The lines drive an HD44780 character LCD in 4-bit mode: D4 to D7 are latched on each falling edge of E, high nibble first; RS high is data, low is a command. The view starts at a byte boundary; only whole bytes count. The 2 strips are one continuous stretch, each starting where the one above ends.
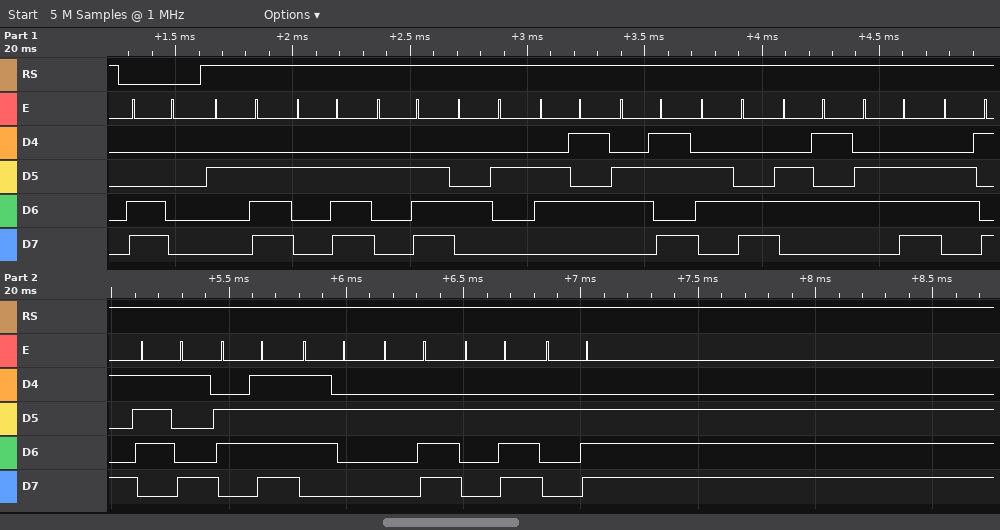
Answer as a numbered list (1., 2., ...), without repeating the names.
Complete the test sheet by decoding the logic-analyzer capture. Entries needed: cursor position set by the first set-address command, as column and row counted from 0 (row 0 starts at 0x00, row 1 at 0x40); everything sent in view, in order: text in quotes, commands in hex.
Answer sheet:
1. column 0, row 1
2. 0xC0 "...Bekleniyor..."
